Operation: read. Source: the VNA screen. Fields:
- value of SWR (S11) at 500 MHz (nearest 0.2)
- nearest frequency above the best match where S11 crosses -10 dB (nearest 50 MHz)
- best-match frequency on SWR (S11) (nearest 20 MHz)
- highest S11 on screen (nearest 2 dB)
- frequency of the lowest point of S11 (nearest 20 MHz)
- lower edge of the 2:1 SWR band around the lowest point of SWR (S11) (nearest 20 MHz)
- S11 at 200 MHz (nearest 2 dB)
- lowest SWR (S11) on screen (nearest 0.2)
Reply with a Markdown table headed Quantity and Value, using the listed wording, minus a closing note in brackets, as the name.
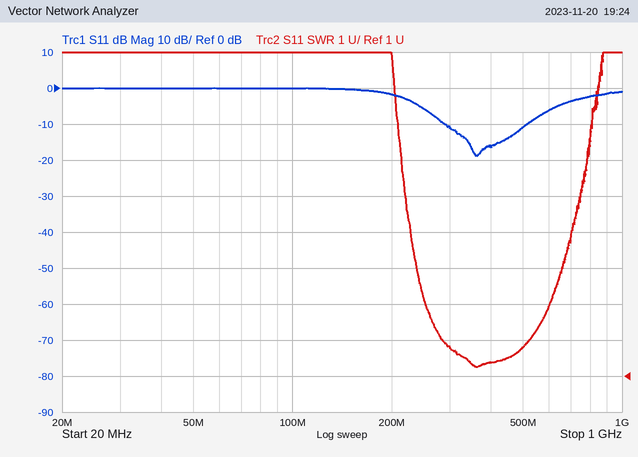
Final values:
| Quantity | Value |
|---|---|
| value of SWR (S11) at 500 MHz | 1.8 |
| nearest frequency above the best match where S11 crosses -10 dB | 500 MHz |
| best-match frequency on SWR (S11) | 360 MHz |
| highest S11 on screen | 0 dB |
| frequency of the lowest point of S11 | 360 MHz |
| lower edge of the 2:1 SWR band around the lowest point of SWR (S11) | 280 MHz |
| S11 at 200 MHz | -2 dB |
| lowest SWR (S11) on screen | 1.2 |
